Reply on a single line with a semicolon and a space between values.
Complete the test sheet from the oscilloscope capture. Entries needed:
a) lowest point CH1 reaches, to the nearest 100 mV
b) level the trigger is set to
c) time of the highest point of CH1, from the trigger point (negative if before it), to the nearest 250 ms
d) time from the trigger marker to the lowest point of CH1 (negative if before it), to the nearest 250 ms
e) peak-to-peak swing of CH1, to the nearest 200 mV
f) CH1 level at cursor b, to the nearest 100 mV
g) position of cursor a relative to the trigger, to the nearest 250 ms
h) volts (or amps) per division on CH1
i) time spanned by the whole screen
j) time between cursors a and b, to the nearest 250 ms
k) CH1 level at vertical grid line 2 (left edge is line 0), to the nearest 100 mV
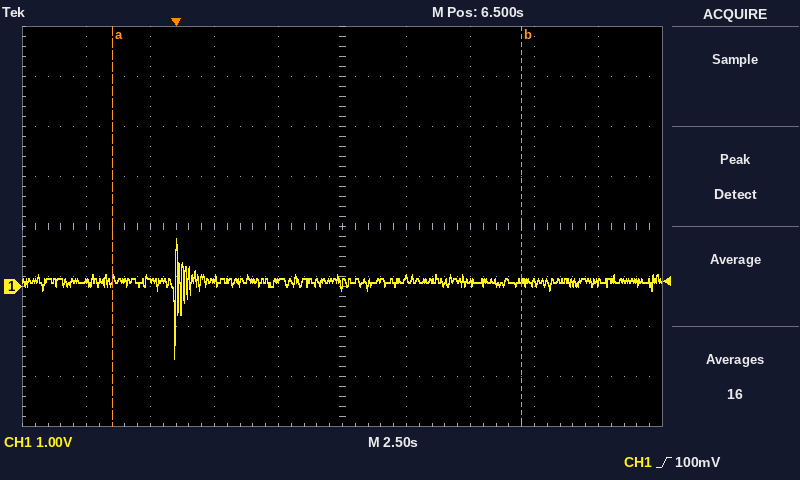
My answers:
-1.4 V; 100 mV; 0.00 s; 0.00 s; 2.4 V; 100 mV; -2.50 s; 1 V; 25 s; 16.00 s; 100 mV
